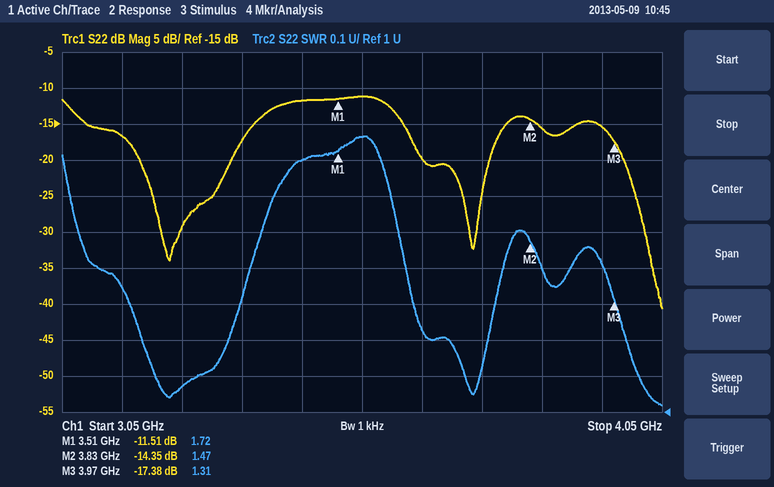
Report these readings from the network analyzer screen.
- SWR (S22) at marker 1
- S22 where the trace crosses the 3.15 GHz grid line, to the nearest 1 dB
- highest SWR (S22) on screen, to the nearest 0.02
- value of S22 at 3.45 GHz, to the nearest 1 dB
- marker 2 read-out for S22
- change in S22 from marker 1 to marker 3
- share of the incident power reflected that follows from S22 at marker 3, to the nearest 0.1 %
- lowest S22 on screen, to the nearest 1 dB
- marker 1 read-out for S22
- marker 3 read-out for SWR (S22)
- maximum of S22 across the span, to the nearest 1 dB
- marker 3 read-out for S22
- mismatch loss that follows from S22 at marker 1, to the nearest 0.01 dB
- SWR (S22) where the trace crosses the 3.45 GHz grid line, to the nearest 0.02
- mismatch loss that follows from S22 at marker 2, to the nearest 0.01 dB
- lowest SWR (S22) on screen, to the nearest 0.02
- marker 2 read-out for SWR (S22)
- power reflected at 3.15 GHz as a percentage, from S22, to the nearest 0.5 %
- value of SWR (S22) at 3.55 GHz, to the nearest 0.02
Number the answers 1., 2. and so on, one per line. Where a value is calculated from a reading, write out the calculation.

1. 1.72
2. -17 dB
3. 1.76
4. -12 dB
5. -14.35 dB
6. -17.38 − (-11.51) = -5.87 dB
7. 10^(-17.38/10) ≈ 1.8 %
8. -41 dB
9. -11.51 dB
10. 1.31
11. -11 dB
12. -17.38 dB
13. −10 log10(1 − 10^(-11.51/10)) ≈ 0.32 dB
14. 1.70
15. −10 log10(1 − 10^(-14.35/10)) ≈ 0.16 dB
16. 1.02
17. 1.47
18. 10^(-17/10) ≈ 2.0 %
19. 1.76
